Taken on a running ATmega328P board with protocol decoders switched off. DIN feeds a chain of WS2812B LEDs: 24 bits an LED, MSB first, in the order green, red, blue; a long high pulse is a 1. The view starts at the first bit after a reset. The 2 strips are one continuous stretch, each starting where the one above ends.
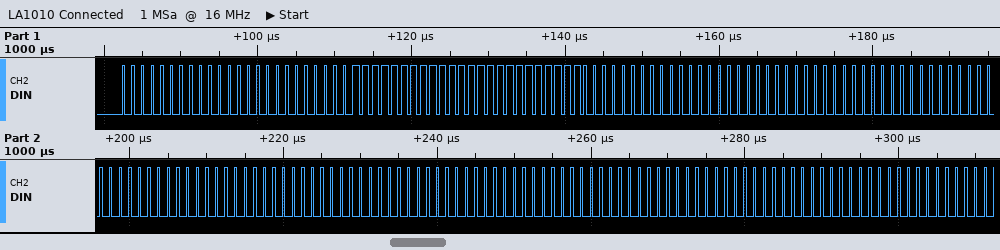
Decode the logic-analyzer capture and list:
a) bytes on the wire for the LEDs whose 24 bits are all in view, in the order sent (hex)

00 00 00 FF FF FF 00 00 00 00 00 00 00 00 00 00 00 00 00 00 00
